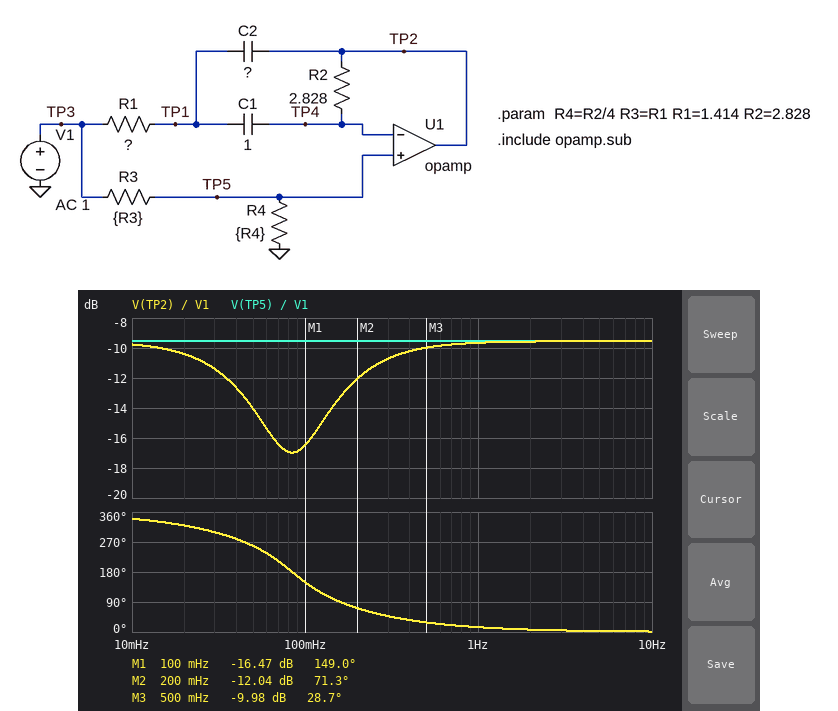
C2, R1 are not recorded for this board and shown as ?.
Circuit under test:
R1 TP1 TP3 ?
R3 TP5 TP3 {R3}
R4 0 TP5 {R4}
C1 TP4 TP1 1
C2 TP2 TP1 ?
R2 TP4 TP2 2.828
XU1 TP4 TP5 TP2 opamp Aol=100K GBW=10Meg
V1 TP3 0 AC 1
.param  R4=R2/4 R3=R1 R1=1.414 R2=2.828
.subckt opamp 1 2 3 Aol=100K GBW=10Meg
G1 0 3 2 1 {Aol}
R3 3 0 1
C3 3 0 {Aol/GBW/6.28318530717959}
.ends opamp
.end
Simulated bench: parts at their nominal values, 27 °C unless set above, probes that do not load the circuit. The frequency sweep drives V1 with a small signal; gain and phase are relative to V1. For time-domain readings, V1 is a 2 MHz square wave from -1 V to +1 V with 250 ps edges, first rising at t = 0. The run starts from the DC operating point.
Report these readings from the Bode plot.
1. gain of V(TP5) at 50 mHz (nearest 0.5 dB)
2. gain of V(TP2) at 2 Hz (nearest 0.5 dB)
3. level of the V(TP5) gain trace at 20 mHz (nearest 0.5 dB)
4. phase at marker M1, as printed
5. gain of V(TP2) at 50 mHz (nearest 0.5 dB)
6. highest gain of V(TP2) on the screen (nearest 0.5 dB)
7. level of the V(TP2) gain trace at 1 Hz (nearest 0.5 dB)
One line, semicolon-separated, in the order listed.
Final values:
-9.5 dB; -9.5 dB; -9.5 dB; 149.0 deg; -14.0 dB; -9.5 dB; -9.5 dB
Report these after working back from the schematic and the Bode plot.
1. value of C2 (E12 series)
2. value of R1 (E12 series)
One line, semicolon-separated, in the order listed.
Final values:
470 mF; 2.7 Ω
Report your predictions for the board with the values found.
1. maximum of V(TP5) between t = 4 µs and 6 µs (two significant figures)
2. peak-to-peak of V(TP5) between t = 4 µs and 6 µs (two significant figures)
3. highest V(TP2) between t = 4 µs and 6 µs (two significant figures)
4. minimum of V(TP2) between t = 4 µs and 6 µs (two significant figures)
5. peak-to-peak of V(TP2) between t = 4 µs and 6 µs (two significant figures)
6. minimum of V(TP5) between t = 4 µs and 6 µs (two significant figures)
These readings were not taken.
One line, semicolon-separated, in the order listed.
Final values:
330 mV; 670 mV; 330 mV; -330 mV; 670 mV; -330 mV
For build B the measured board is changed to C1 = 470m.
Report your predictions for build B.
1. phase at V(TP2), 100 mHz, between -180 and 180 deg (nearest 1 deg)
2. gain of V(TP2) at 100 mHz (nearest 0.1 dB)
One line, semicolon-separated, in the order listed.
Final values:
-91 deg; -23.1 dB
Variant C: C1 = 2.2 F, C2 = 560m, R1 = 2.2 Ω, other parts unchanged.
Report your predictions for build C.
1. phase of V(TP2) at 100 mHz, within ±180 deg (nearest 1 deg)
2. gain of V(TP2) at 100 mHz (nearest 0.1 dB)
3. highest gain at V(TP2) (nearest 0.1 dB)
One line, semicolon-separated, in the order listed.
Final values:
125 deg; -9.2 dB; -9.1 dB
